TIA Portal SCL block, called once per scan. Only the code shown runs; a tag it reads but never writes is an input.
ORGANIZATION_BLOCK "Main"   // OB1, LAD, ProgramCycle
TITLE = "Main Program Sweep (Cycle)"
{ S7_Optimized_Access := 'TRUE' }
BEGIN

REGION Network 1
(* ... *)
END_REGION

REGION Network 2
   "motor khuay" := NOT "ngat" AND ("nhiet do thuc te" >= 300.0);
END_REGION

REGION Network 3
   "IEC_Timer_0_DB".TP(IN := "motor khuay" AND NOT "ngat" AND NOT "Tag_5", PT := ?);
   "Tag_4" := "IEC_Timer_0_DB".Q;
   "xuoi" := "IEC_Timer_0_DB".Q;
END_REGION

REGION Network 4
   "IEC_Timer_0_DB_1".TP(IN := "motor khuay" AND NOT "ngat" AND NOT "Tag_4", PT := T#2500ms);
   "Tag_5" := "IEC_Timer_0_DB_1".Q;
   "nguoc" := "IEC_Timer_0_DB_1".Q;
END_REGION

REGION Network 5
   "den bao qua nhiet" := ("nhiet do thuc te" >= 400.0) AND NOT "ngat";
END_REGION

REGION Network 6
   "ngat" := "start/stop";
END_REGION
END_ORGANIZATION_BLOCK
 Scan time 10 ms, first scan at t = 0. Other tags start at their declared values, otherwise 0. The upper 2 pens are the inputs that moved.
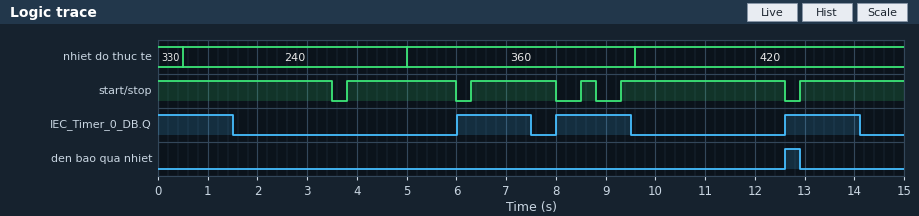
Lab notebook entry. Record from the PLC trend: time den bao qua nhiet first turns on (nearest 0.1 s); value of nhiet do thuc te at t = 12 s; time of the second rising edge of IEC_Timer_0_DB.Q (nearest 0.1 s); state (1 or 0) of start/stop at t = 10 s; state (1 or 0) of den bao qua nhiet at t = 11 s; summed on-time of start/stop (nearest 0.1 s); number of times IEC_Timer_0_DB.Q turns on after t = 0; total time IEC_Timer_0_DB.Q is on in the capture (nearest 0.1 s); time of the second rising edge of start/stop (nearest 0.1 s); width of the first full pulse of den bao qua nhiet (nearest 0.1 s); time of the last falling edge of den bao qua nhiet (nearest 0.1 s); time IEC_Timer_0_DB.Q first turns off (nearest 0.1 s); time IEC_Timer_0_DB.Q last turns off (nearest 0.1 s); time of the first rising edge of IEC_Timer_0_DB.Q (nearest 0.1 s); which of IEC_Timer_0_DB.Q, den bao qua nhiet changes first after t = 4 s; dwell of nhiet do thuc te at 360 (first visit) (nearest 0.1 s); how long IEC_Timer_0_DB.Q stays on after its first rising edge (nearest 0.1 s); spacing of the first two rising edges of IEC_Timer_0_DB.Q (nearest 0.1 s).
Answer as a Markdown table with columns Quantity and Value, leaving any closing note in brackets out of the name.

| Quantity | Value |
|---|---|
| time den bao qua nhiet first turns on | 12.6 s |
| value of nhiet do thuc te at t = 12 s | 420 |
| time of the second rising edge of IEC_Timer_0_DB.Q | 8.0 s |
| state (1 or 0) of start/stop at t = 10 s | 1 |
| state (1 or 0) of den bao qua nhiet at t = 11 s | 0 |
| summed on-time of start/stop | 13.1 s |
| number of times IEC_Timer_0_DB.Q turns on after t = 0 | 3 |
| total time IEC_Timer_0_DB.Q is on in the capture | 6.0 s |
| time of the second rising edge of start/stop | 6.3 s |
| width of the first full pulse of den bao qua nhiet | 0.3 s |
| time of the last falling edge of den bao qua nhiet | 12.9 s |
| time IEC_Timer_0_DB.Q first turns off | 1.5 s |
| time IEC_Timer_0_DB.Q last turns off | 14.1 s |
| time of the first rising edge of IEC_Timer_0_DB.Q | 6.0 s |
| which of IEC_Timer_0_DB.Q, den bao qua nhiet changes first after t = 4 s | IEC_Timer_0_DB.Q |
| dwell of nhiet do thuc te at 360 (first visit) | 4.6 s |
| how long IEC_Timer_0_DB.Q stays on after its first rising edge | 1.5 s |
| spacing of the first two rising edges of IEC_Timer_0_DB.Q | 2.0 s |
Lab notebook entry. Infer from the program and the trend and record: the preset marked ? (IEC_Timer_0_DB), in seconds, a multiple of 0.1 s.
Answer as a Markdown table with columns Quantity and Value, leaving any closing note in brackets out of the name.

| Quantity | Value |
|---|---|
| the preset marked ? (IEC_Timer_0_DB), in seconds, a multiple of 0.1 s | 1.5 s |
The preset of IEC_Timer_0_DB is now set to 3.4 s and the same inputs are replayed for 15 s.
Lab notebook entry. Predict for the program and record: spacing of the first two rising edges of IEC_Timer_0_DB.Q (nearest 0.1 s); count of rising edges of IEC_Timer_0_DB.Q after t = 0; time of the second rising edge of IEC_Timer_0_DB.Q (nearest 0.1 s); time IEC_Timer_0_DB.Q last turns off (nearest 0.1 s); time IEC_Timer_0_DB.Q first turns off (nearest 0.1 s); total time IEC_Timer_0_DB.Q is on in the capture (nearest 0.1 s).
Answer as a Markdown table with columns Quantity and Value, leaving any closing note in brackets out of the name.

| Quantity | Value |
|---|---|
| spacing of the first two rising edges of IEC_Timer_0_DB.Q | 6.6 s |
| count of rising edges of IEC_Timer_0_DB.Q after t = 0 | 2 |
| time of the second rising edge of IEC_Timer_0_DB.Q | 12.6 s |
| time IEC_Timer_0_DB.Q last turns off | 9.4 s |
| time IEC_Timer_0_DB.Q first turns off | 3.4 s |
| total time IEC_Timer_0_DB.Q is on in the capture | 9.2 s |
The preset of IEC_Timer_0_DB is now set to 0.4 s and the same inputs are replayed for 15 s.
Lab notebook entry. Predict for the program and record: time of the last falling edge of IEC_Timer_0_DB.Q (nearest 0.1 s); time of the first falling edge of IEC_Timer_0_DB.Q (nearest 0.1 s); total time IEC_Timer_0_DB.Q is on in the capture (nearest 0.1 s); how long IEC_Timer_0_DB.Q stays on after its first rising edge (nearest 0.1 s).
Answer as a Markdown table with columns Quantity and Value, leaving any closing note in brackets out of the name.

| Quantity | Value |
|---|---|
| time of the last falling edge of IEC_Timer_0_DB.Q | 13.0 s |
| time of the first falling edge of IEC_Timer_0_DB.Q | 0.4 s |
| total time IEC_Timer_0_DB.Q is on in the capture | 1.6 s |
| how long IEC_Timer_0_DB.Q stays on after its first rising edge | 0.4 s |
